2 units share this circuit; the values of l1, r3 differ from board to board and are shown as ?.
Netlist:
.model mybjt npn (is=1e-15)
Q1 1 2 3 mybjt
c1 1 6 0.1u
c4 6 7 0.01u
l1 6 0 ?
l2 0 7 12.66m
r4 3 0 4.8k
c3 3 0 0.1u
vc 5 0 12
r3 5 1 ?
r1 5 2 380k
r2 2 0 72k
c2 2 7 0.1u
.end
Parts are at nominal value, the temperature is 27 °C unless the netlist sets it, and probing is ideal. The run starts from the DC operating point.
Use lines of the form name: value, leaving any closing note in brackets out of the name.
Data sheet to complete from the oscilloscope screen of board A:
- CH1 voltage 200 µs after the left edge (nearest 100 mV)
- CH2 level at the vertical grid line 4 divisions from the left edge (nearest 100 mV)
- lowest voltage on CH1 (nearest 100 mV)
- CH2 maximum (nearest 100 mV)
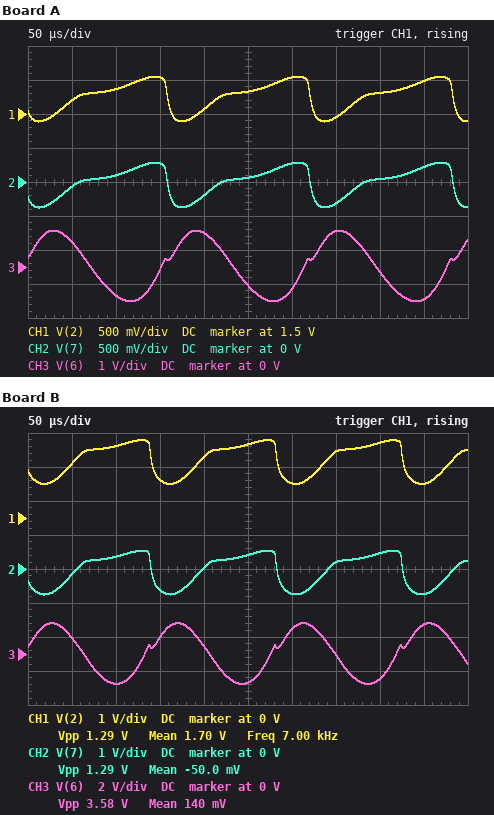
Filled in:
CH1 voltage 200 µs after the left edge: 1.6 V
CH2 level at the vertical grid line 4 divisions from the left edge: -200 mV
lowest voltage on CH1: 1.4 V
CH2 maximum: 300 mV
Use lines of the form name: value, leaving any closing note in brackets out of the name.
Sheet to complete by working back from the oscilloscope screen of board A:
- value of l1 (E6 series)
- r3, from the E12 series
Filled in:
value of l1: 47 mH
r3, from the E12 series: 2.7 kΩ
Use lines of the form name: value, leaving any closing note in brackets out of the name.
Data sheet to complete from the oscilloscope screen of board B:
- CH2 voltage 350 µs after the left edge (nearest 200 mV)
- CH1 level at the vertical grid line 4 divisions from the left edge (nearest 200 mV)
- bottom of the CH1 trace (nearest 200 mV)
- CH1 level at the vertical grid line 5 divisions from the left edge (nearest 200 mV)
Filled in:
CH2 voltage 350 µs after the left edge: 200 mV
CH1 level at the vertical grid line 4 divisions from the left edge: 1.8 V
bottom of the CH1 trace: 1.0 V
CH1 level at the vertical grid line 5 divisions from the left edge: 2.2 V
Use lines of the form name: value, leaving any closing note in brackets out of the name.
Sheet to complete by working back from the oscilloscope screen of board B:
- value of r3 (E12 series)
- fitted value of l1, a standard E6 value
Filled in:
value of r3: 3.9 kΩ
fitted value of l1, a standard E6 value: 33 mH
